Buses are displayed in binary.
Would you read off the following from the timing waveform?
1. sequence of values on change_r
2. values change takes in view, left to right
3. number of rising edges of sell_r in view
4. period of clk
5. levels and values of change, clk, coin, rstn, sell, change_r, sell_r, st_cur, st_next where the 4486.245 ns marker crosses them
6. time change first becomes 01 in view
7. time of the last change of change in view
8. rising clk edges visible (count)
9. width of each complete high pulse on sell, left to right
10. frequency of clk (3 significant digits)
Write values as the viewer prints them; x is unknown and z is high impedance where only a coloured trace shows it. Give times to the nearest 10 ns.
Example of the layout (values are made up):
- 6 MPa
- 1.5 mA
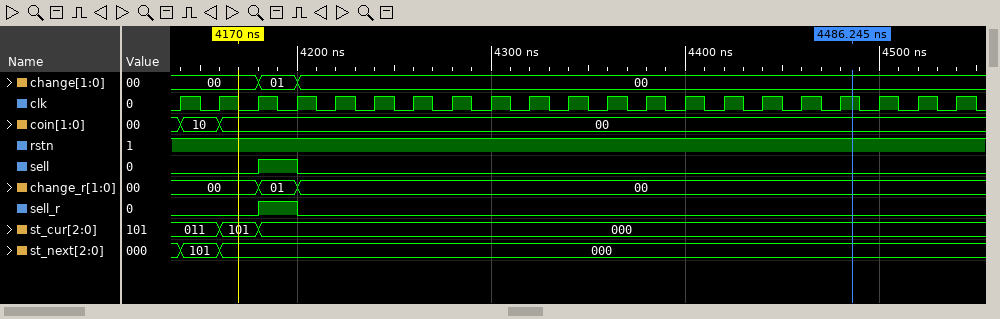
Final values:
- 00, 01, 00
- 00, 01, 00
- 1
- 20 ns
- change=00, clk=1, coin=00, rstn=1, sell=0, change_r=00, sell_r=0, st_cur=000, st_next=000
- 4180 ns
- 4200 ns
- 21
- 20 ns
- 50.0 MHz
